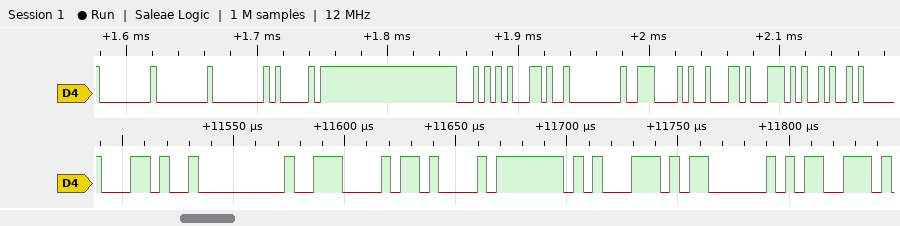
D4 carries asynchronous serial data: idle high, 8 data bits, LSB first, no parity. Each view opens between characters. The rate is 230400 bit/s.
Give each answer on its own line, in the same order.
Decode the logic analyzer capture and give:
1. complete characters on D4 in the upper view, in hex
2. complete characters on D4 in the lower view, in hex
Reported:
00, 00, 00, 41, 54, 2C, 00, 0E, 89, 71, 29
2C, 00, 0E, 0B, 7F, 71, 03, CD
